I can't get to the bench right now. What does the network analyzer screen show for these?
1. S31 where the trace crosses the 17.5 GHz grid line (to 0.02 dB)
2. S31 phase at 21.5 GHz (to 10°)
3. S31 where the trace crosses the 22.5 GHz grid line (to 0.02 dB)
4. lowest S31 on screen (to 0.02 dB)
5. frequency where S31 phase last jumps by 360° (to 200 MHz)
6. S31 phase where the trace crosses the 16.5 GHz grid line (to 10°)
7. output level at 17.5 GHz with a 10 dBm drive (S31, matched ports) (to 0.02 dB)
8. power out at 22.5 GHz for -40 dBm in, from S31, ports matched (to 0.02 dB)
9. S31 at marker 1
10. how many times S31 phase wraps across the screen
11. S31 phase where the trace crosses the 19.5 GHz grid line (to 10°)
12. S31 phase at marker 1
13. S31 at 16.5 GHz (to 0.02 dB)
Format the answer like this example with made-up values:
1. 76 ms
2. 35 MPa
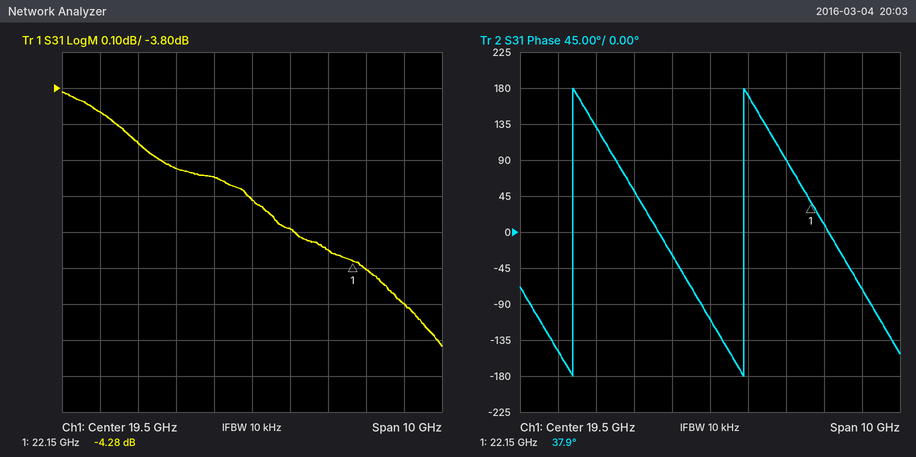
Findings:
1. -4.02 dB
2. 90°
3. -4.30 dB
4. -4.52 dB
5. 20.4 GHz
6. 130°
7. 5.98 dBm
8. -44.30 dBm
9. -4.28 dB
10. 2
11. -110°
12. 37.9°
13. -3.96 dB
